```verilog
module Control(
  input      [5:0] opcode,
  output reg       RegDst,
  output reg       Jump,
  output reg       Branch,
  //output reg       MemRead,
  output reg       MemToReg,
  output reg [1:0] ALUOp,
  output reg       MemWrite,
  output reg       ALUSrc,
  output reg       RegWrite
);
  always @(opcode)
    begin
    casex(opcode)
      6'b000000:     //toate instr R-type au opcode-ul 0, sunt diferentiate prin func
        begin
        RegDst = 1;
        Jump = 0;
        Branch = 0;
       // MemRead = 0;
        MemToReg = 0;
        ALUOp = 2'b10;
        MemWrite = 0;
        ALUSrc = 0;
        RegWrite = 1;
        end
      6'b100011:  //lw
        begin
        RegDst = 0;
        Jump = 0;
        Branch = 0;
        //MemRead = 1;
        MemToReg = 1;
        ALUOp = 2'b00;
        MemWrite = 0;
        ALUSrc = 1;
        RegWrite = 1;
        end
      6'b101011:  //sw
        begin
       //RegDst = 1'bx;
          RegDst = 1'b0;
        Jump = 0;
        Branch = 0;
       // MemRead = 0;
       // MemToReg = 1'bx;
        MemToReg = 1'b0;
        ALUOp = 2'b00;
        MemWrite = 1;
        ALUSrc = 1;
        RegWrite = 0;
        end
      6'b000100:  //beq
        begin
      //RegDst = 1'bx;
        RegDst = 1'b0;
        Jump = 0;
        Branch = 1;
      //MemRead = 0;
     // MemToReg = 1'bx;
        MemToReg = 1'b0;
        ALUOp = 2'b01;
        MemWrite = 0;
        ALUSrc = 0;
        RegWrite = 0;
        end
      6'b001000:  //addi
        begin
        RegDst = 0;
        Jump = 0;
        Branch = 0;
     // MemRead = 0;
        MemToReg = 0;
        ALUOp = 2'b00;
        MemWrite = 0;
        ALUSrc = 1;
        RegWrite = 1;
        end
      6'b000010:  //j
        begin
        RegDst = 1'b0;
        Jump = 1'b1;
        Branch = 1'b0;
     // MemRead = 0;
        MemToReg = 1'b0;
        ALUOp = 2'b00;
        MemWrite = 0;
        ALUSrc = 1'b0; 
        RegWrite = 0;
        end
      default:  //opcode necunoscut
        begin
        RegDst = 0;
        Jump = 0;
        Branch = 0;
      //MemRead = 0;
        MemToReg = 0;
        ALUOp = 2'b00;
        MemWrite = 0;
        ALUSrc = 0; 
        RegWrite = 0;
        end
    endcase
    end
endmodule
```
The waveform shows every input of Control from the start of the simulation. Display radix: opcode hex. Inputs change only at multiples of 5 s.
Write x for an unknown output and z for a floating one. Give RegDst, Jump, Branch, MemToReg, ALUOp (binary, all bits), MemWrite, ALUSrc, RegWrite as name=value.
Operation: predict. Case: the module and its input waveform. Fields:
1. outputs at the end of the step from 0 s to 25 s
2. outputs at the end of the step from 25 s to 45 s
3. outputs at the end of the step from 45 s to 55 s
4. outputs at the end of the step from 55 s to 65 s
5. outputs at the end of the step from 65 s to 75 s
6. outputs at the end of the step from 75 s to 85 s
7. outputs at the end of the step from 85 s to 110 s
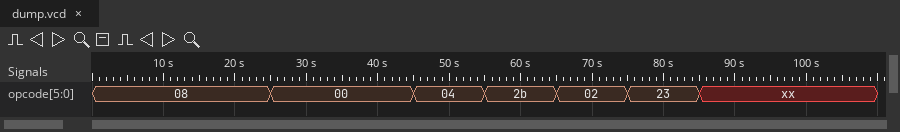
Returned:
RegDst=0, Jump=0, Branch=0, MemToReg=0, ALUOp=00, MemWrite=0, ALUSrc=1, RegWrite=1
RegDst=1, Jump=0, Branch=0, MemToReg=0, ALUOp=10, MemWrite=0, ALUSrc=0, RegWrite=1
RegDst=0, Jump=0, Branch=1, MemToReg=0, ALUOp=01, MemWrite=0, ALUSrc=0, RegWrite=0
RegDst=0, Jump=0, Branch=0, MemToReg=0, ALUOp=00, MemWrite=1, ALUSrc=1, RegWrite=0
RegDst=0, Jump=1, Branch=0, MemToReg=0, ALUOp=00, MemWrite=0, ALUSrc=0, RegWrite=0
RegDst=0, Jump=0, Branch=0, MemToReg=1, ALUOp=00, MemWrite=0, ALUSrc=1, RegWrite=1
RegDst=1, Jump=0, Branch=0, MemToReg=0, ALUOp=10, MemWrite=0, ALUSrc=0, RegWrite=1
